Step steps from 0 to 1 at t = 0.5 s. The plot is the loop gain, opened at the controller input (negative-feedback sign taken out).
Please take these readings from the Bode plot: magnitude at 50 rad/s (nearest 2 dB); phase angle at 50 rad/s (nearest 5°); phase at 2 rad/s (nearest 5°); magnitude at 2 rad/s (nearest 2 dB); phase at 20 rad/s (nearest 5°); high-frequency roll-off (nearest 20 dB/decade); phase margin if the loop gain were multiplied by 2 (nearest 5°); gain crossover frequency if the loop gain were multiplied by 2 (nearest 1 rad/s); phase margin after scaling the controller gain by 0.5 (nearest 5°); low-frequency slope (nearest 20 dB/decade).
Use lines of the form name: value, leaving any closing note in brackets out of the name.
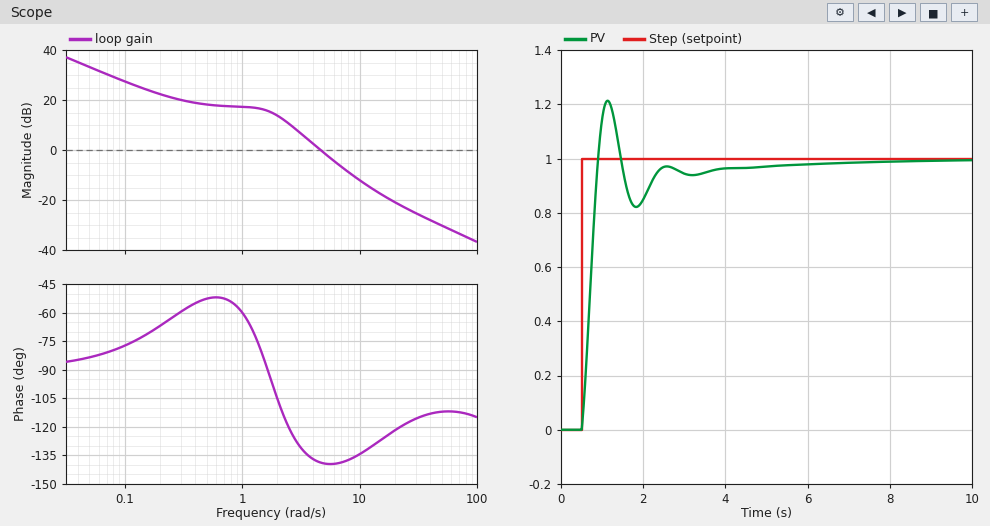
magnitude at 50 rad/s: -30 dB
phase angle at 50 rad/s: -110°
phase at 2 rad/s: -105°
magnitude at 2 rad/s: 14 dB
phase at 20 rad/s: -120°
high-frequency roll-off: -20 dB/decade
phase margin if the loop gain were multiplied by 2: 40°
gain crossover frequency if the loop gain were multiplied by 2: 7 rad/s
phase margin after scaling the controller gain by 0.5: 50°
low-frequency slope: -20 dB/decade
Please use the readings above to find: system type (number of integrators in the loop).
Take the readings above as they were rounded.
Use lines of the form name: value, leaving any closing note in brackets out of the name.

system type: 1
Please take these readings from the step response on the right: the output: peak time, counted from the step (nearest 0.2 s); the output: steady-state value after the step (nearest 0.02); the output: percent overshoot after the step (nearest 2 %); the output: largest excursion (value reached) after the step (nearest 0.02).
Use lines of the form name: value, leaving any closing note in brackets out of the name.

the output: peak time, counted from the step: 0.6 s
the output: steady-state value after the step: 1.00
the output: percent overshoot after the step: 22 %
the output: largest excursion (value reached) after the step: 1.22
